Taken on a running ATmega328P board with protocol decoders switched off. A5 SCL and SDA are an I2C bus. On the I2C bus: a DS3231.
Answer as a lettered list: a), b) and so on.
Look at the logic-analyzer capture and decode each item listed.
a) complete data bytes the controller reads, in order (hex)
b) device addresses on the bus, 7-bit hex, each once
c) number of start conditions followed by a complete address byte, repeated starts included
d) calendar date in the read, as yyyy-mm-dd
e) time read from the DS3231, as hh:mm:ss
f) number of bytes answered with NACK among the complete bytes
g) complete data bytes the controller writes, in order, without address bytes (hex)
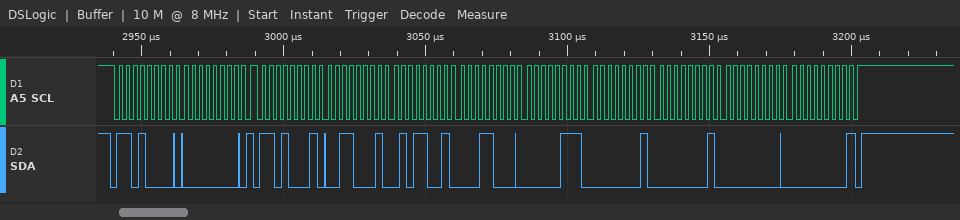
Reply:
a) 31 59 18 07 01 01 00 00
b) 0x68
c) 2
d) 2000-01-01
e) 18:59:31
f) 1
g) 00
